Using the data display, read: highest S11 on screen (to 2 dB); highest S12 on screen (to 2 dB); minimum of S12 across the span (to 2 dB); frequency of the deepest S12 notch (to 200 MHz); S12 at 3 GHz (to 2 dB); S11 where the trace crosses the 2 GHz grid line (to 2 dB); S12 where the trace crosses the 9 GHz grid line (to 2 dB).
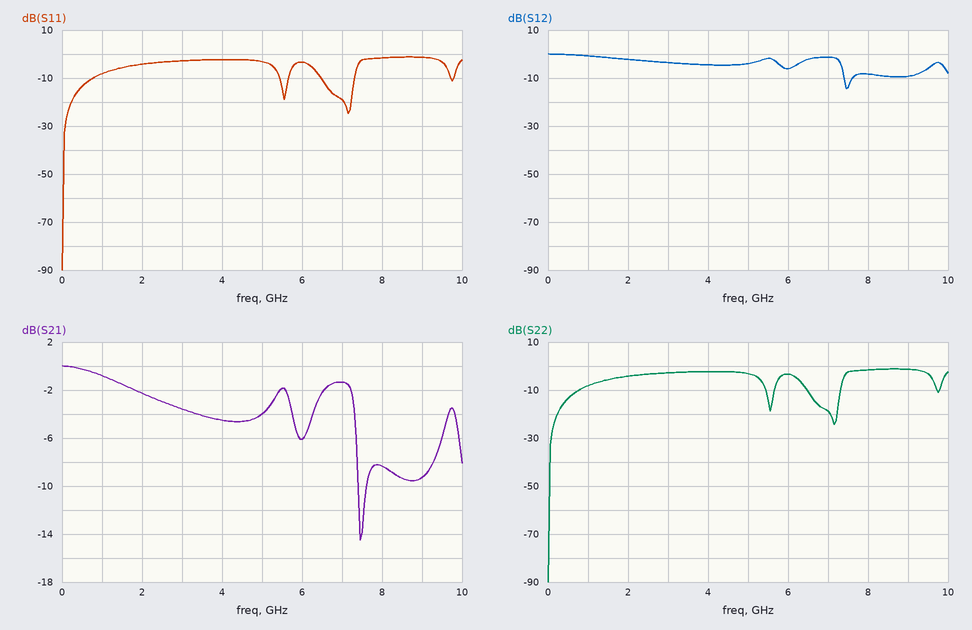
-2 dB
0 dB
-14 dB
7.4 GHz
-4 dB
-4 dB
-10 dB
